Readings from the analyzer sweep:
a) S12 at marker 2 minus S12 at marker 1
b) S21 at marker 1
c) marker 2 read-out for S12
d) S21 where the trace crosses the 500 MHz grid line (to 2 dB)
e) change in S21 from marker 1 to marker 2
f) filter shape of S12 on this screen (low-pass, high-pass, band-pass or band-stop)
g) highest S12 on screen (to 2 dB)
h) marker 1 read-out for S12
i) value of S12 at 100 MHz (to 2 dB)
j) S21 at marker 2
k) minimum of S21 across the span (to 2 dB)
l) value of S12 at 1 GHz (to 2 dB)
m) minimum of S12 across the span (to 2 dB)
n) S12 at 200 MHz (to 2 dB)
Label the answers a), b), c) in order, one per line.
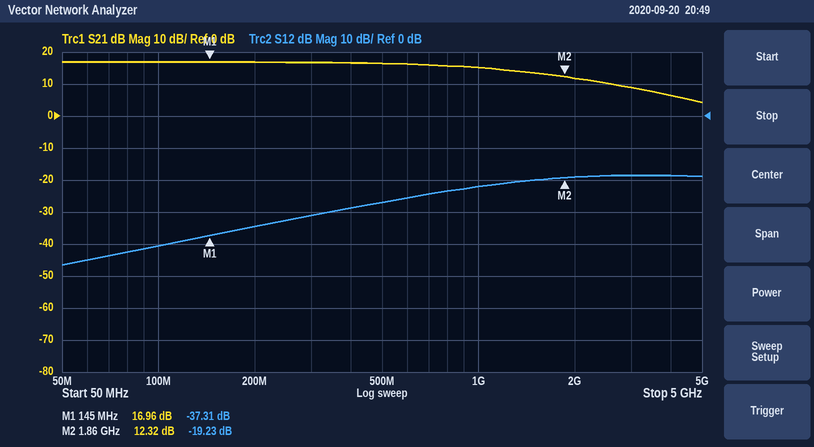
a) 18.08 dB
b) 16.96 dB
c) -19.23 dB
d) 16 dB
e) -4.64 dB
f) high-pass
g) -18 dB
h) -37.31 dB
i) -40 dB
j) 12.32 dB
k) 4 dB
l) -22 dB
m) -46 dB
n) -34 dB
